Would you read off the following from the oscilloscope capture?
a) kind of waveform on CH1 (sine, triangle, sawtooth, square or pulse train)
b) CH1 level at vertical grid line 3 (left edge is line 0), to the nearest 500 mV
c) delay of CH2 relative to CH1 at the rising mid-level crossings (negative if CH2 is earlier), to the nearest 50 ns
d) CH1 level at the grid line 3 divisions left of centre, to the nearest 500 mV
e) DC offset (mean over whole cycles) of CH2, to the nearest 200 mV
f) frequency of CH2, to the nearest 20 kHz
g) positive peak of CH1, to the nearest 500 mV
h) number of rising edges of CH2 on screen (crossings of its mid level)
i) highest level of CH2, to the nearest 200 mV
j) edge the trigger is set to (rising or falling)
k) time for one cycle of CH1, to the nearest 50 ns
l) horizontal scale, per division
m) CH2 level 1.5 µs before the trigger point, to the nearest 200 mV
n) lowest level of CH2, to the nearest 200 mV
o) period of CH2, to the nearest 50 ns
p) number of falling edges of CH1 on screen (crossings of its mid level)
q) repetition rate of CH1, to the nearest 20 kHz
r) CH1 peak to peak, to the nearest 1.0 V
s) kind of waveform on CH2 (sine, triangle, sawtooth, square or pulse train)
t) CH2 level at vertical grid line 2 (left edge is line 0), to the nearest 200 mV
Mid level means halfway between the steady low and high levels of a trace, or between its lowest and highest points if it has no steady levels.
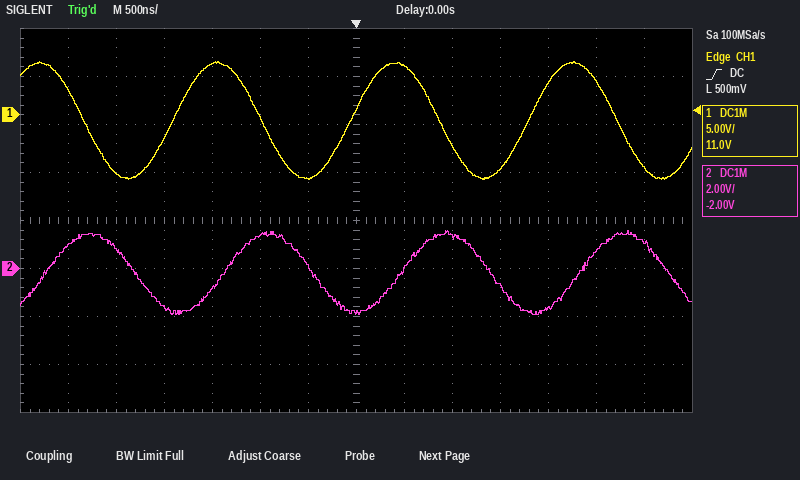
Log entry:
sine
-2.5 V
+550 ns
5.5 V
-200 mV
540 kHz
5.5 V
4
1.6 V
rising
1.85 µs
500 ns
-800 mV
-2.0 V
1.85 µs
4
540 kHz
12.0 V
sine
800 mV
